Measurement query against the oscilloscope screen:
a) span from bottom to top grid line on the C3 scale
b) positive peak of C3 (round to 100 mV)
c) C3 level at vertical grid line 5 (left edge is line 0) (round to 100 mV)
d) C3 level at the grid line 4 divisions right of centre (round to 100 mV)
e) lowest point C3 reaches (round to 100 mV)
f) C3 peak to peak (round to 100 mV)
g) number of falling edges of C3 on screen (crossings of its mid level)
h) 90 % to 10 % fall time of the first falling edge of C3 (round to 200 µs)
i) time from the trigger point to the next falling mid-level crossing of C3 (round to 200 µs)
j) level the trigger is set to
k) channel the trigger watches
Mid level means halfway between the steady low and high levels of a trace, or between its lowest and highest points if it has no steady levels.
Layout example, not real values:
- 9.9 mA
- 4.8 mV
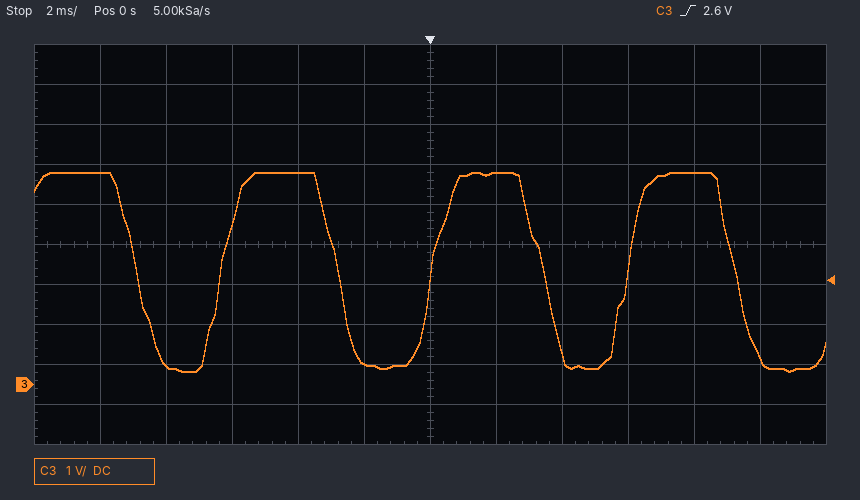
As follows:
- 10 V
- 5.3 V
- 500 mV
- 5.3 V
- 300 mV
- 5.0 V
- 4
- 1.2 ms
- 3.4 ms
- 2.6 V
- C3
